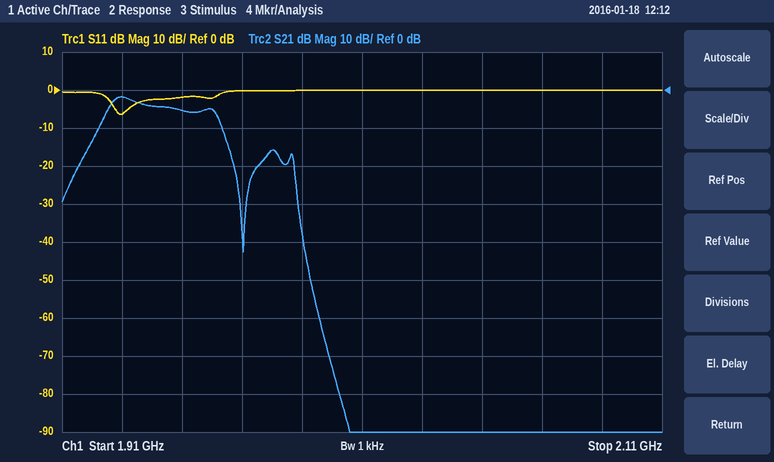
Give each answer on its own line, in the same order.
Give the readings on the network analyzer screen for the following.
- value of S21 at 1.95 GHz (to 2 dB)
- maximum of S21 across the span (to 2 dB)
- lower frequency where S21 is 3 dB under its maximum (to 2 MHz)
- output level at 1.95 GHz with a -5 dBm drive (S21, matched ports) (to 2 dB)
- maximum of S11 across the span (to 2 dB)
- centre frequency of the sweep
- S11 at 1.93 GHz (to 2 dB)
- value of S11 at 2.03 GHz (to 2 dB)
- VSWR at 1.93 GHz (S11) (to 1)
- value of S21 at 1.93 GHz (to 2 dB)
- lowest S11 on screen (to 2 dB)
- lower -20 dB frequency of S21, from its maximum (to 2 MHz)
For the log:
-6 dB
-2 dB
1.926 GHz
-10 dBm
0 dB
2.01 GHz
-6 dB
0 dB
3
-2 dB
-6 dB
1.914 GHz
